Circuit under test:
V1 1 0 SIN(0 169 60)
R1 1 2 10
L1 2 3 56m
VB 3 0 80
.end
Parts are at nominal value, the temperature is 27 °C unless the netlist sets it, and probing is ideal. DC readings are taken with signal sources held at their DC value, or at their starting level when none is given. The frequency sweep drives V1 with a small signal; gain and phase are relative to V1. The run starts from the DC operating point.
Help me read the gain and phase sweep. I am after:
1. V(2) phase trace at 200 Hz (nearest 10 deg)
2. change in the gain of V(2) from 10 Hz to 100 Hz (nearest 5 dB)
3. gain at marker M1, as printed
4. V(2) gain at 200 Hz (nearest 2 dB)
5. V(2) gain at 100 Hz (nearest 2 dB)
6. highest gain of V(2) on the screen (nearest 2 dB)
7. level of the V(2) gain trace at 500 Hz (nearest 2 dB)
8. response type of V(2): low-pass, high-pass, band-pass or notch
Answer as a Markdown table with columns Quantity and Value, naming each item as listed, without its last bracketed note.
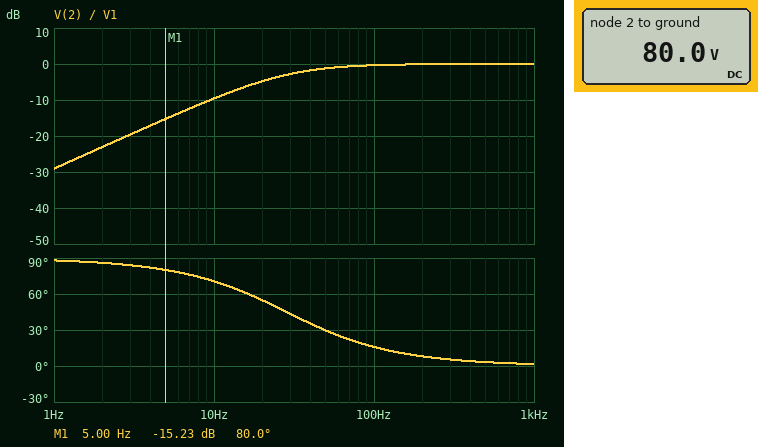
| Quantity | Value |
|---|---|
| V(2) phase trace at 200 Hz | 10 deg |
| change in the gain of V(2) from 10 Hz to 100 Hz | 10 dB |
| gain at marker M1, as printed | -15.23 dB |
| V(2) gain at 200 Hz | 0 dB |
| V(2) gain at 100 Hz | 0 dB |
| highest gain of V(2) on the screen | 0 dB |
| level of the V(2) gain trace at 500 Hz | 0 dB |
| response type of V(2): low-pass, high-pass, band-pass or notch | high-pass |
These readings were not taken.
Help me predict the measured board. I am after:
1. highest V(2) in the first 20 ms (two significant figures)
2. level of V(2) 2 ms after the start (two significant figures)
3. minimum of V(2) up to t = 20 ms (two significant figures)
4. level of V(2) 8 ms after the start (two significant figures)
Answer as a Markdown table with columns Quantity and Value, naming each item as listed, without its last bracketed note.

| Quantity | Value |
|---|---|
| highest V(2) in the first 20 ms | 230 V |
| level of V(2) 2 ms after the start | 180 V |
| minimum of V(2) up to t = 20 ms | -81 V |
| level of V(2) 8 ms after the start | 17 V |
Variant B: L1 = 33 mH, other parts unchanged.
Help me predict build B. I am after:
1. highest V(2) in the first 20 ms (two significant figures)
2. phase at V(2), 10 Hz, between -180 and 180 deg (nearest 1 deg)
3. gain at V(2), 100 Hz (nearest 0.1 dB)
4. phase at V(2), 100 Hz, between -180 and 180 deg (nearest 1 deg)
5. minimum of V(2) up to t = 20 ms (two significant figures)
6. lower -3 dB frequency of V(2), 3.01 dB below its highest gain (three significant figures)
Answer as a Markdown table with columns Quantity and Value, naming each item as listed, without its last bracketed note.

| Quantity | Value |
|---|---|
| highest V(2) in the first 20 ms | 210 V |
| phase at V(2), 10 Hz, between -180 and 180 deg | 78 deg |
| gain at V(2), 100 Hz | -0.9 dB |
| phase at V(2), 100 Hz, between -180 and 180 deg | 26 deg |
| minimum of V(2) up to t = 20 ms | -55 V |
| lower -3 dB frequency of V(2), 3.01 dB below its highest gain | 48.2 Hz |
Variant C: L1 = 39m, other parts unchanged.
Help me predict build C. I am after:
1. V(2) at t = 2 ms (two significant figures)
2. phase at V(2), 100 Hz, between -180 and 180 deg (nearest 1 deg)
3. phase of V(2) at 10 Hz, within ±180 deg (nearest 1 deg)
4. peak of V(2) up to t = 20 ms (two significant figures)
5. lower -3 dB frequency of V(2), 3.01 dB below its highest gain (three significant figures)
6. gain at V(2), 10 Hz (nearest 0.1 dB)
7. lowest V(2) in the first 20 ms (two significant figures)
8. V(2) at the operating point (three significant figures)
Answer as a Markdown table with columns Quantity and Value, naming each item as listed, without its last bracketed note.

| Quantity | Value |
|---|---|
| V(2) at t = 2 ms | 170 V |
| phase at V(2), 100 Hz, between -180 and 180 deg | 22 deg |
| phase of V(2) at 10 Hz, within ±180 deg | 76 deg |
| peak of V(2) up to t = 20 ms | 220 V |
| lower -3 dB frequency of V(2), 3.01 dB below its highest gain | 40.8 Hz |
| gain at V(2), 10 Hz | -12.5 dB |
| lowest V(2) in the first 20 ms | -65 V |
| V(2) at the operating point | 80.0 V |
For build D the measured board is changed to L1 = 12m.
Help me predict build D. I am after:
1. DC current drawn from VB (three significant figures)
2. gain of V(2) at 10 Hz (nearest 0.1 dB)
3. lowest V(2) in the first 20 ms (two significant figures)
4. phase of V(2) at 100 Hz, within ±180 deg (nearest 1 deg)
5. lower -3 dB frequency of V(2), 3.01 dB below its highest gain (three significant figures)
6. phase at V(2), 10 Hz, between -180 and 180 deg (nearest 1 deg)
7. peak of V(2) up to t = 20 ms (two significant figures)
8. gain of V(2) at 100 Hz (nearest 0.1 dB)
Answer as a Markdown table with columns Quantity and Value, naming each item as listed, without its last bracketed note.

| Quantity | Value |
|---|---|
| DC current drawn from VB | 8.00 A |
| gain of V(2) at 10 Hz | -22.5 dB |
| lowest V(2) in the first 20 ms | 10 V |
| phase of V(2) at 100 Hz, within ±180 deg | 53 deg |
| lower -3 dB frequency of V(2), 3.01 dB below its highest gain | 133 Hz |
| phase at V(2), 10 Hz, between -180 and 180 deg | 86 deg |
| peak of V(2) up to t = 20 ms | 150 V |
| gain of V(2) at 100 Hz | -4.4 dB |
